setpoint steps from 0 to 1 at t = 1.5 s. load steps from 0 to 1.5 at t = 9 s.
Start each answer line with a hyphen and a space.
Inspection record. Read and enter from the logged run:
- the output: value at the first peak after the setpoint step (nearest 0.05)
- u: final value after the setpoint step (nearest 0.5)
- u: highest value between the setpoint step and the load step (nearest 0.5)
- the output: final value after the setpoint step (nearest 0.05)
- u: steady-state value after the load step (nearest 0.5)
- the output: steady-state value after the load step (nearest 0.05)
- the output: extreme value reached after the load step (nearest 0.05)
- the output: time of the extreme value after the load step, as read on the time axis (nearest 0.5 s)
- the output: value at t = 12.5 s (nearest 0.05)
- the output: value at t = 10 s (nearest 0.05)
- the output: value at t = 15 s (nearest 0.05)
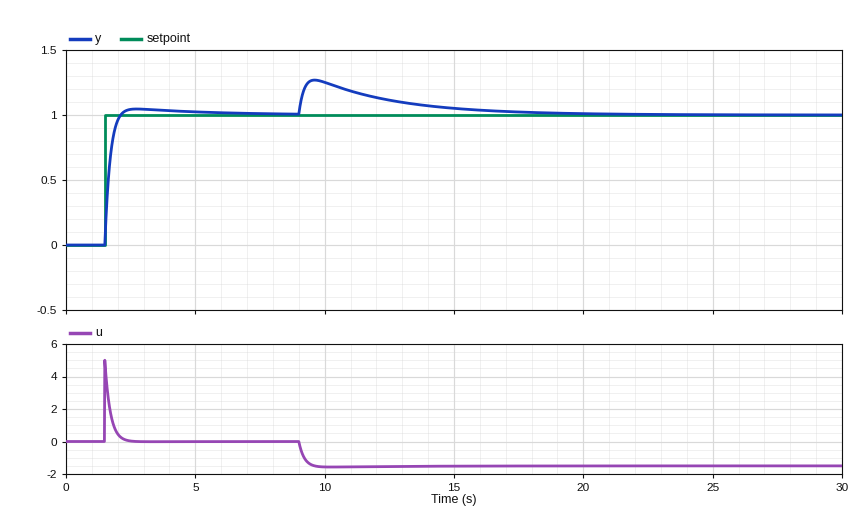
- 1.05
- 0.0
- 5.0
- 1.00
- -1.5
- 1.00
- 1.25
- 9.5 s
- 1.10
- 1.25
- 1.05
